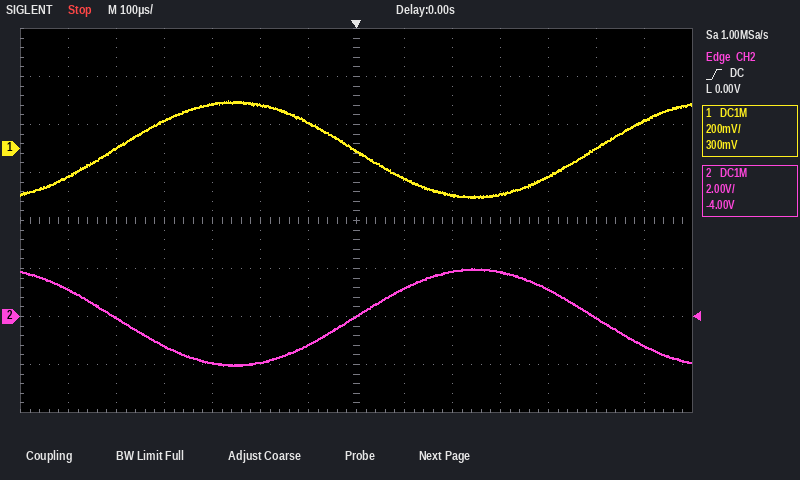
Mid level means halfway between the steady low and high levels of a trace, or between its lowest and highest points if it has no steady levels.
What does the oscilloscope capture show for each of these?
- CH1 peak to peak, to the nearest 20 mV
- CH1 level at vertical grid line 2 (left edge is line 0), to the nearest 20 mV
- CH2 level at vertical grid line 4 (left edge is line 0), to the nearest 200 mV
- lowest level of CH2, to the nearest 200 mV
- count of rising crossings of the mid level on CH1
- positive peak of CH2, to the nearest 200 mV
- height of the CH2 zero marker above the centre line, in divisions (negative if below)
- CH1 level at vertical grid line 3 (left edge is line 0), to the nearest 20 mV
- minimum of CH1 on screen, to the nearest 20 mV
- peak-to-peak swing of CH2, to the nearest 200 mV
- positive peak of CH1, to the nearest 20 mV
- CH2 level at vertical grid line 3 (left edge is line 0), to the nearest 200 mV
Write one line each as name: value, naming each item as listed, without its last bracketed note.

CH1 peak to peak, to the nearest 20 mV: 400 mV
CH1 level at vertical grid line 2 (left edge is line 0), to the nearest 20 mV: 0 mV
CH2 level at vertical grid line 4 (left edge is line 0), to the nearest 200 mV: -2.0 V
lowest level of CH2, to the nearest 200 mV: -2.0 V
count of rising crossings of the mid level on CH1: 2
positive peak of CH2, to the nearest 200 mV: 2.0 V
height of the CH2 zero marker above the centre line, in divisions: -2.0 div
CH1 level at vertical grid line 3 (left edge is line 0), to the nearest 20 mV: 120 mV
minimum of CH1 on screen, to the nearest 20 mV: -200 mV
peak-to-peak swing of CH2, to the nearest 200 mV: 4.0 V
positive peak of CH1, to the nearest 20 mV: 200 mV
CH2 level at vertical grid line 3 (left edge is line 0), to the nearest 200 mV: -1.2 V
